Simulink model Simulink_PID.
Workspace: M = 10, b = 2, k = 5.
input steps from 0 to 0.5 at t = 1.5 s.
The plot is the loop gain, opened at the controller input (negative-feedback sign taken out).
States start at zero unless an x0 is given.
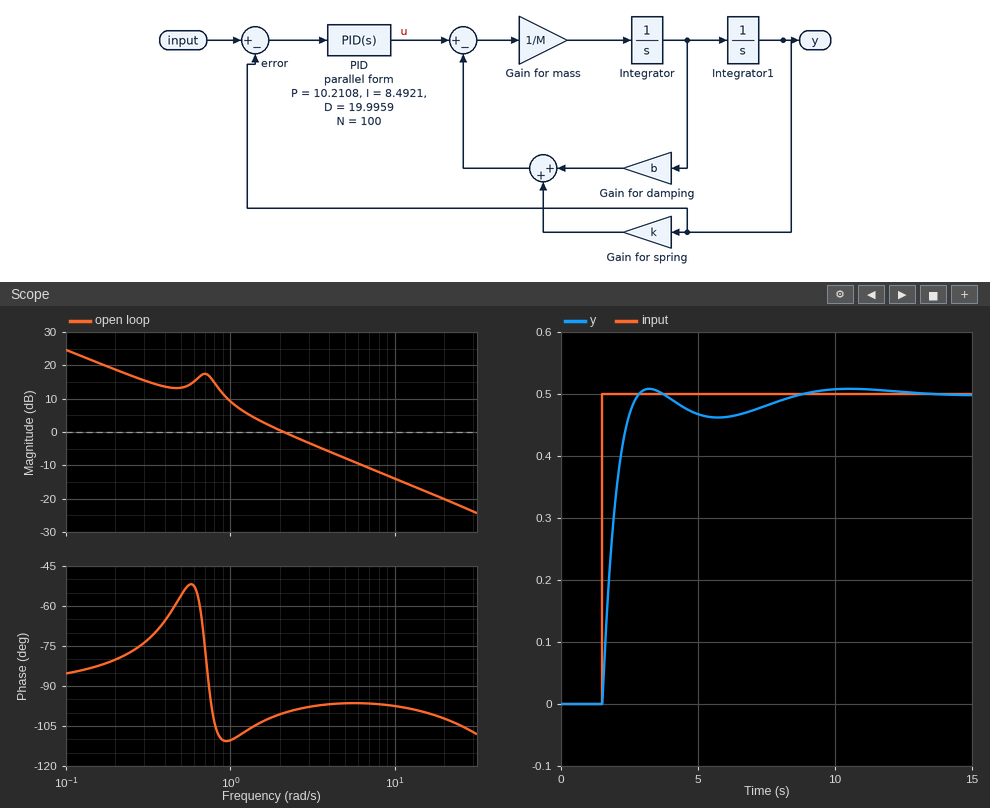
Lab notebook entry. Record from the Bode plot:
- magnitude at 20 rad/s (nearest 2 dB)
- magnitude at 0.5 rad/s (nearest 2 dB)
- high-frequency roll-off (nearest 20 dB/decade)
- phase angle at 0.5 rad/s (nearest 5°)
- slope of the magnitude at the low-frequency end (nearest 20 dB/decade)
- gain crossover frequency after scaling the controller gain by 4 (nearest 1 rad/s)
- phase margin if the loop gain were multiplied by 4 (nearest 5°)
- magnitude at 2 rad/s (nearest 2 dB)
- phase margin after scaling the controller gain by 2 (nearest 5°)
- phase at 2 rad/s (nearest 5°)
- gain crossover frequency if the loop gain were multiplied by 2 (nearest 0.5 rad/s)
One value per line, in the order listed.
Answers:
-20 dB
14 dB
-20 dB/decade
-55°
-20 dB/decade
8 rad/s
85°
0 dB
85°
-100°
4.0 rad/s
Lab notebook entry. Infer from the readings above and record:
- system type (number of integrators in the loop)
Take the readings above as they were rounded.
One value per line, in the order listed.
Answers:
1
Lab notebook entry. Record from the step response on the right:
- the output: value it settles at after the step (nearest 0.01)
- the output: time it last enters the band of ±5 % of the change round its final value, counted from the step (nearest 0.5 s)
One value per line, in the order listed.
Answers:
0.50
5.5 s
